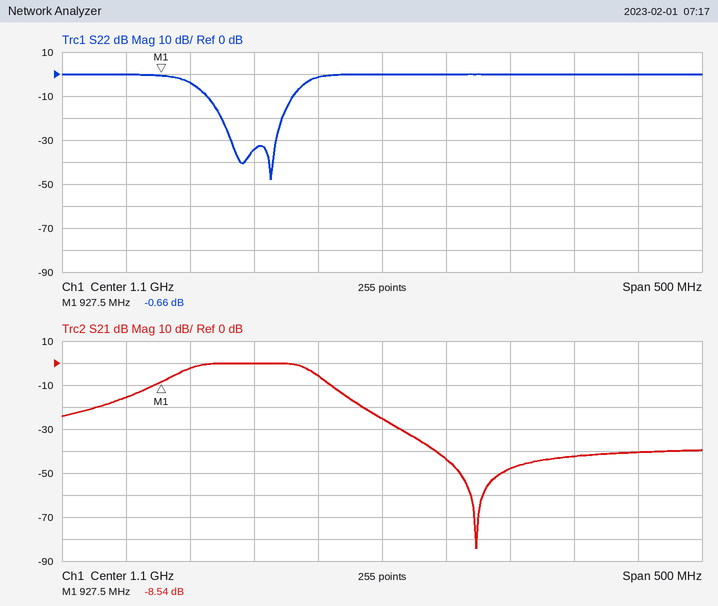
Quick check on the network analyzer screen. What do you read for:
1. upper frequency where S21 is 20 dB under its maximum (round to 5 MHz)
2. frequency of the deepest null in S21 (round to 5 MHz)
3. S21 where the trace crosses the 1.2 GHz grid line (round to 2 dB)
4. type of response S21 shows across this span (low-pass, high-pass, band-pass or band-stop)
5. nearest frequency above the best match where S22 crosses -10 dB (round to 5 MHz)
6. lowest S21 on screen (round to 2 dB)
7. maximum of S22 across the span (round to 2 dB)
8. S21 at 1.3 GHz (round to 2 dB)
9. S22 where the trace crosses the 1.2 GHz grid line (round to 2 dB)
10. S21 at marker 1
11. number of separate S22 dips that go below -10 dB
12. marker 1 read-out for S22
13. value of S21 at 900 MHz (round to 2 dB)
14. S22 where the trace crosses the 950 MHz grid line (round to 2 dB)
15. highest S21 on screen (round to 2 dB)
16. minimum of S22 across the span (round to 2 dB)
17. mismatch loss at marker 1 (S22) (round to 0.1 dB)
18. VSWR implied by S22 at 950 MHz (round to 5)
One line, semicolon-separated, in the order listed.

1.085 GHz; 1.175 GHz; -48 dB; band-pass; 1.030 GHz; -84 dB; 0 dB; -40 dB; 0 dB; -8.54 dB; 2; -0.66 dB; -16 dB; -4 dB; 0 dB; -48 dB; 8.5 dB; 5
